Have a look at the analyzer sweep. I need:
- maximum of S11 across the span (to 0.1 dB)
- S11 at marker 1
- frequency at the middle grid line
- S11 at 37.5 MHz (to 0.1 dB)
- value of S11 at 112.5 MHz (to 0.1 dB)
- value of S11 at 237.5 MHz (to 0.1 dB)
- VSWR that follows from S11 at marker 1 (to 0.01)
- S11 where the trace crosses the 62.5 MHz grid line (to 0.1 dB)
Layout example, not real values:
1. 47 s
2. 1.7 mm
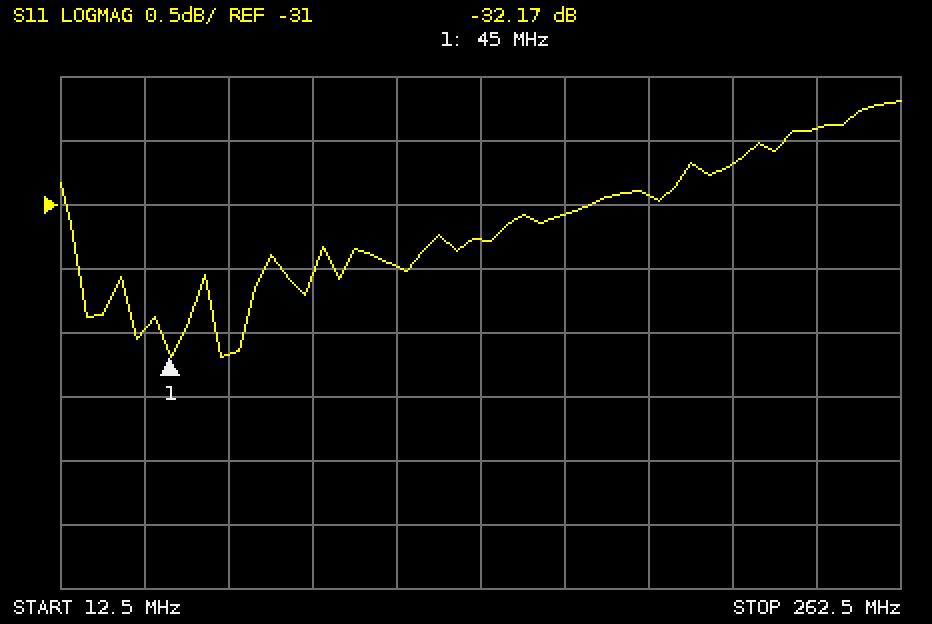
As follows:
1. -30.2 dB
2. -32.17 dB
3. 137.5 MHz
4. -32.0 dB
5. -31.5 dB
6. -30.4 dB
7. 1.05
8. -32.2 dB
